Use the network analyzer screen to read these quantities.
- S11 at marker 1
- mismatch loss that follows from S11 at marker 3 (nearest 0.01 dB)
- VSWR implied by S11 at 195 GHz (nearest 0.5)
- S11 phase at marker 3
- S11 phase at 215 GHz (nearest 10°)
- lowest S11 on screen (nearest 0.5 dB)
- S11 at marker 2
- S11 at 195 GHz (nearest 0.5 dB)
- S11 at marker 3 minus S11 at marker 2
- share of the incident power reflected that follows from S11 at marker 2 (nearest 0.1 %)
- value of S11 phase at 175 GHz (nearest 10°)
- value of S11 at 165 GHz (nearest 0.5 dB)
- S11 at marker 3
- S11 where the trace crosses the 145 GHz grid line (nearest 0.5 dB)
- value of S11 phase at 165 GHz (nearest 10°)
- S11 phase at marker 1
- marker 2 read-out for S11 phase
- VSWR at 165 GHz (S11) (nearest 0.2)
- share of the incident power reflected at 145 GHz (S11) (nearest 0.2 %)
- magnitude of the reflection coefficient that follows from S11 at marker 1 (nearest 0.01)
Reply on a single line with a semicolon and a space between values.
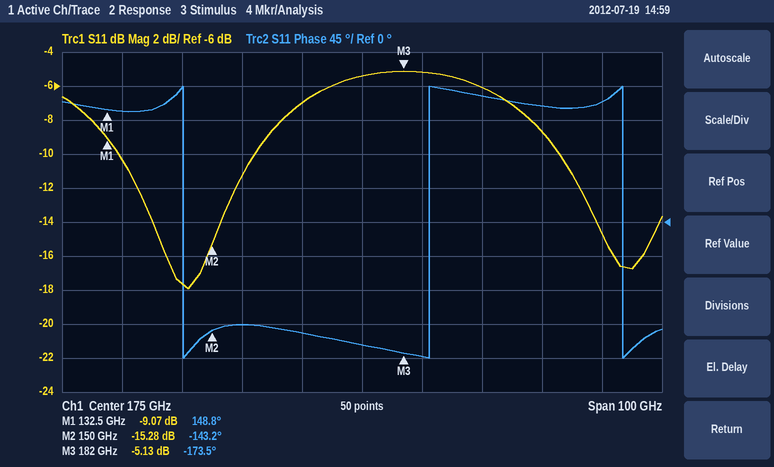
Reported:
-9.07 dB; 1.59 dB; 3.0; -173.5°; 160°; -18.0 dB; -15.28 dB; -6.0 dB; 10.15 dB; 3.0 %; -160°; -7.0 dB; -5.13 dB; -17.5 dB; -150°; 148.8°; -143.2°; 2.6; 1.8 %; 0.35
